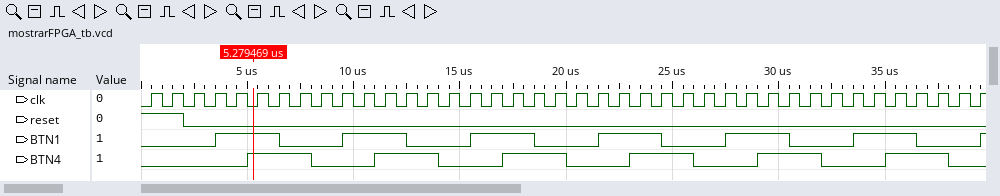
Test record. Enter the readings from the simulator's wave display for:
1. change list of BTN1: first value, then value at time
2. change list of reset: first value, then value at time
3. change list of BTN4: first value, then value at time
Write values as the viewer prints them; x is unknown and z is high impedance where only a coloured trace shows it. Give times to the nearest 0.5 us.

0, 1 at 3.5 us, 0 at 6.5 us, 1 at 9.5 us, 0 at 12.5 us, 1 at 15.5 us, 0 at 18.5 us, 1 at 21.5 us, 0 at 24.5 us, 1 at 27.5 us, 0 at 30.5 us, 1 at 33.5 us, 0 at 36.5 us, 1 at 39.5 us
1, 0 at 2 us
0, 1 at 5 us, 0 at 8 us, 1 at 11 us, 0 at 14 us, 1 at 17 us, 0 at 20 us, 1 at 23 us, 0 at 26 us, 1 at 29 us, 0 at 32 us, 1 at 35 us, 0 at 38 us
